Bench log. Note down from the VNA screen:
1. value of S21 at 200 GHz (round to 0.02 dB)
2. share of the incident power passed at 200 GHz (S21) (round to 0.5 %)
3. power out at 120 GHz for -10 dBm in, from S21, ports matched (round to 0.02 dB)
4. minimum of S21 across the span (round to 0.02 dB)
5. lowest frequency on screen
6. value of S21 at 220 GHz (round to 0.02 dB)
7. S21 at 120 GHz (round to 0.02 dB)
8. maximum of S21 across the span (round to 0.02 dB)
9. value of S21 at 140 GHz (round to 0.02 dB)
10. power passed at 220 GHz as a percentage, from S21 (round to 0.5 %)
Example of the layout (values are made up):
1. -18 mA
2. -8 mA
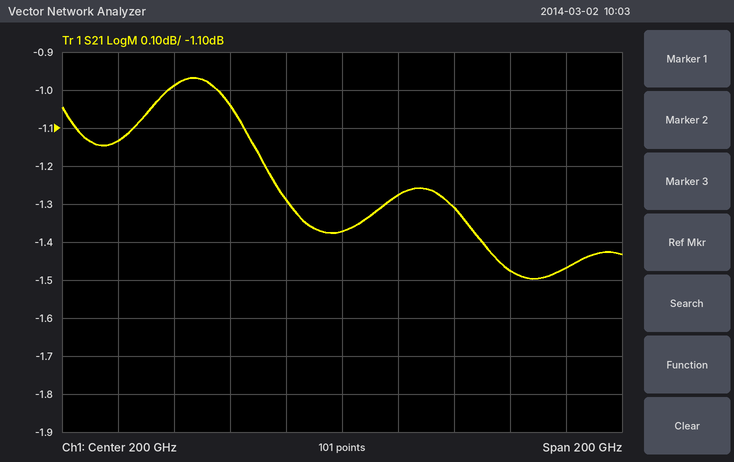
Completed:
1. -1.38 dB
2. 73.0 %
3. -11.14 dBm
4. -1.50 dB
5. 100 GHz
6. -1.28 dB
7. -1.14 dB
8. -0.96 dB
9. -0.98 dB
10. 74.5 %
